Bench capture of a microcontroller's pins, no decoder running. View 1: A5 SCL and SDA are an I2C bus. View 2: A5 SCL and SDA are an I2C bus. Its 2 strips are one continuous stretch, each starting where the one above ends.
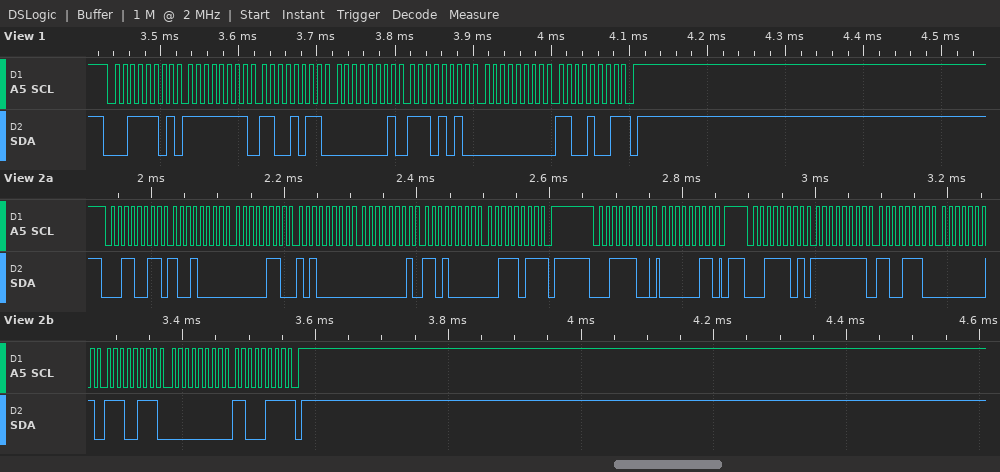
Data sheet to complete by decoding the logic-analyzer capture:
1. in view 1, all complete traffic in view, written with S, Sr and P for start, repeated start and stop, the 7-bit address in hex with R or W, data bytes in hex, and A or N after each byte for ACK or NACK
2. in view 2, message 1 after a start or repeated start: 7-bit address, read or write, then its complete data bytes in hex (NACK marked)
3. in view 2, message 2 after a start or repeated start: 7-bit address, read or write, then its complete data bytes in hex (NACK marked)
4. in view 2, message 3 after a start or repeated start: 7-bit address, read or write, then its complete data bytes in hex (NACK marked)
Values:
S 1ER A FF A CB A 01 A EA A 00 A C9 N P
0x19 read: 90 06 A0 01 D0 3B NACK
0x1E write: 03
0x1E read: FF CE 01 E7 00 C7 NACK
